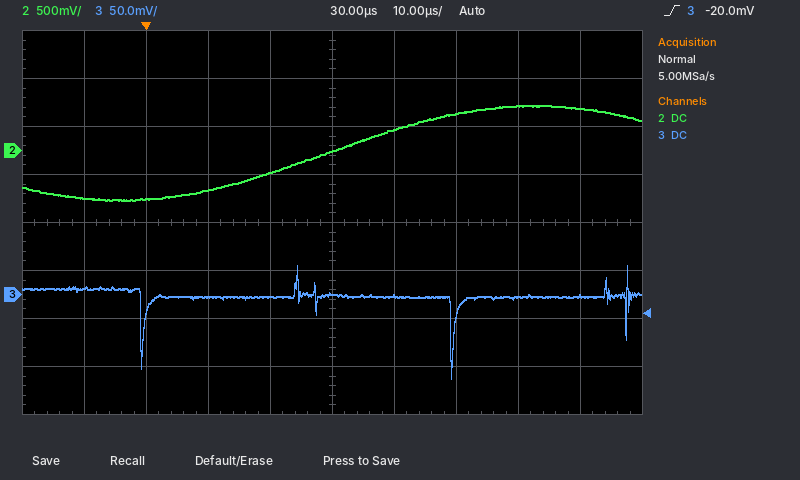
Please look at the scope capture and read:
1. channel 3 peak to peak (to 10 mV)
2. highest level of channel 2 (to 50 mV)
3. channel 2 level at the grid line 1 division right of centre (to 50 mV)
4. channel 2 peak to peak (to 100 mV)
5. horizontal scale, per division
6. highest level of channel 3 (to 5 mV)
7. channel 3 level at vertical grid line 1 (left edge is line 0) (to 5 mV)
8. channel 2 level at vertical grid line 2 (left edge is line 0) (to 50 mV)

120 mV
450 mV
200 mV
1.00 V
10 µs
30 mV
5 mV
-500 mV
